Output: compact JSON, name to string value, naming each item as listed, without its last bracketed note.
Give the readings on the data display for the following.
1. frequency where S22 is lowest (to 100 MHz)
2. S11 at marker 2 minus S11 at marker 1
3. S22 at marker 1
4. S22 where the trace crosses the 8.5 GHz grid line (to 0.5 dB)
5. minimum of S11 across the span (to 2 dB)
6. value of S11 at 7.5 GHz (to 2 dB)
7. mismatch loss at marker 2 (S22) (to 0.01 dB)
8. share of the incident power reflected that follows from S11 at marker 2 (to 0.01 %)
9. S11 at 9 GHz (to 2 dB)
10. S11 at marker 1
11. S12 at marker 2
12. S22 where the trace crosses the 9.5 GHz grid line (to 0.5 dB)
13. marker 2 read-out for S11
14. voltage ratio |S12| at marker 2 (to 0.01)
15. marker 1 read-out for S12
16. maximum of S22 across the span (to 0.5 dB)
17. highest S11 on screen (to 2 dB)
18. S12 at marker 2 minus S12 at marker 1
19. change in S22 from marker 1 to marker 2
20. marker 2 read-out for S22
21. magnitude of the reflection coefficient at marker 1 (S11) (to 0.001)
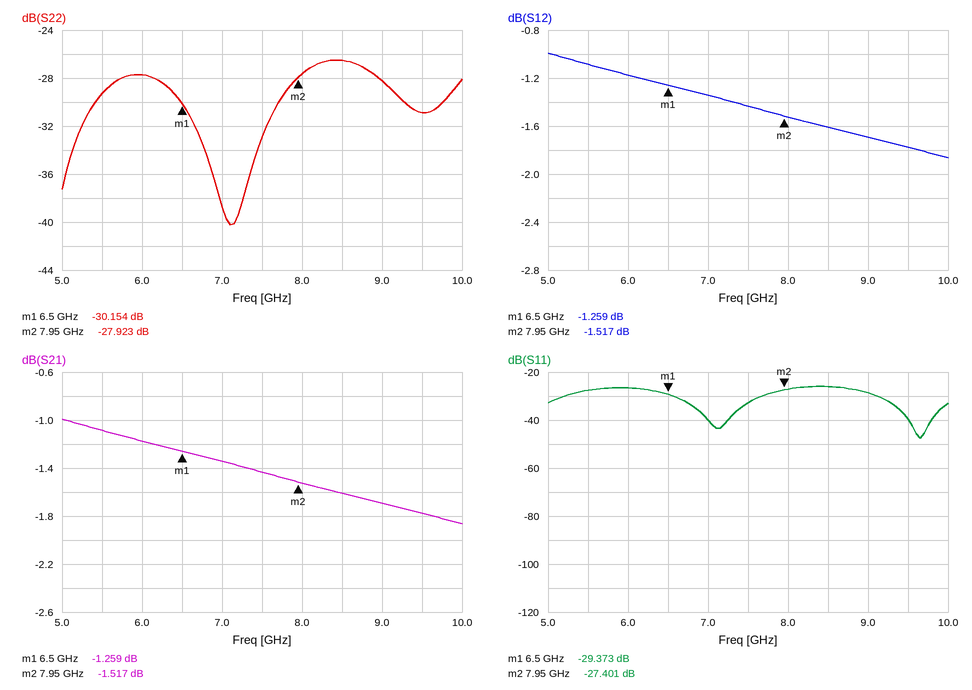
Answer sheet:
{"frequency where S22 is lowest": "7.1 GHz", "S11 at marker 2 minus S11 at marker 1": "1.972 dB", "S22 at marker 1": "-30.154 dB", "S22 where the trace crosses the 8.5 GHz grid line": "-26.5 dB", "minimum of S11 across the span": "-48 dB", "value of S11 at 7.5 GHz": "-32 dB", "mismatch loss at marker 2 (S22)": "0.01 dB", "share of the incident power reflected that follows from S11 at marker 2": "0.18 %", "S11 at 9 GHz": "-28 dB", "S11 at marker 1": "-29.373 dB", "S12 at marker 2": "-1.517 dB", "S22 where the trace crosses the 9.5 GHz grid line": "-31.0 dB", "marker 2 read-out for S11": "-27.401 dB", "voltage ratio |S12| at marker 2": "0.84", "marker 1 read-out for S12": "-1.259 dB", "maximum of S22 across the span": "-26.5 dB", "highest S11 on screen": "-26 dB", "S12 at marker 2 minus S12 at marker 1": "-0.258 dB", "change in S22 from marker 1 to marker 2": "2.231 dB", "marker 2 read-out for S22": "-27.923 dB", "magnitude of the reflection coefficient at marker 1 (S11)": "0.034"}
